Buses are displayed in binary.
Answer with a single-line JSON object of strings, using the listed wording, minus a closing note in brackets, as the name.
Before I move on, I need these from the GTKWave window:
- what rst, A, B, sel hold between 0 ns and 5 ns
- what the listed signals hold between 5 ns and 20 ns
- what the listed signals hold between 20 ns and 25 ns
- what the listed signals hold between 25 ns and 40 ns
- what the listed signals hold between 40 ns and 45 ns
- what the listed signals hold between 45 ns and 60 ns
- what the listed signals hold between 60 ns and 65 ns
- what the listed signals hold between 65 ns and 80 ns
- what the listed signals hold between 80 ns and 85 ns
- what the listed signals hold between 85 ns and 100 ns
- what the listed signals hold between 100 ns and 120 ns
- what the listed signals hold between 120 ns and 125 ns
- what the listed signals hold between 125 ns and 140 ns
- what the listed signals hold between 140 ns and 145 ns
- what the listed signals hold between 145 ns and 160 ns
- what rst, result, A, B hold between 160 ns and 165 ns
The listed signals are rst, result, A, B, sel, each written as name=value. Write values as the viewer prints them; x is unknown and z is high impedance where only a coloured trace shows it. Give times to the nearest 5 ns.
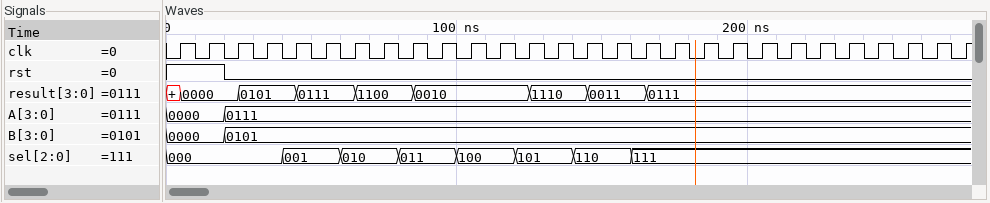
{"what rst, A, B, sel hold between 0 ns and 5 ns": "rst=1, A=0000, B=0000, sel=000", "what the listed signals hold between 5 ns and 20 ns": "rst=1, result=0000, A=0000, B=0000, sel=000", "what the listed signals hold between 20 ns and 25 ns": "rst=0, result=0000, A=0111, B=0101, sel=000", "what the listed signals hold between 25 ns and 40 ns": "rst=0, result=0101, A=0111, B=0101, sel=000", "what the listed signals hold between 40 ns and 45 ns": "rst=0, result=0101, A=0111, B=0101, sel=001", "what the listed signals hold between 45 ns and 60 ns": "rst=0, result=0111, A=0111, B=0101, sel=001", "what the listed signals hold between 60 ns and 65 ns": "rst=0, result=0111, A=0111, B=0101, sel=010", "what the listed signals hold between 65 ns and 80 ns": "rst=0, result=1100, A=0111, B=0101, sel=010", "what the listed signals hold between 80 ns and 85 ns": "rst=0, result=1100, A=0111, B=0101, sel=011", "what the listed signals hold between 85 ns and 100 ns": "rst=0, result=0010, A=0111, B=0101, sel=011", "what the listed signals hold between 100 ns and 120 ns": "rst=0, result=0010, A=0111, B=0101, sel=100", "what the listed signals hold between 120 ns and 125 ns": "rst=0, result=0010, A=0111, B=0101, sel=101", "what the listed signals hold between 125 ns and 140 ns": "rst=0, result=1110, A=0111, B=0101, sel=101", "what the listed signals hold between 140 ns and 145 ns": "rst=0, result=1110, A=0111, B=0101, sel=110", "what the listed signals hold between 145 ns and 160 ns": "rst=0, result=0011, A=0111, B=0101, sel=110", "what rst, result, A, B hold between 160 ns and 165 ns": "rst=0, result=0011, A=0111, B=0101"}
